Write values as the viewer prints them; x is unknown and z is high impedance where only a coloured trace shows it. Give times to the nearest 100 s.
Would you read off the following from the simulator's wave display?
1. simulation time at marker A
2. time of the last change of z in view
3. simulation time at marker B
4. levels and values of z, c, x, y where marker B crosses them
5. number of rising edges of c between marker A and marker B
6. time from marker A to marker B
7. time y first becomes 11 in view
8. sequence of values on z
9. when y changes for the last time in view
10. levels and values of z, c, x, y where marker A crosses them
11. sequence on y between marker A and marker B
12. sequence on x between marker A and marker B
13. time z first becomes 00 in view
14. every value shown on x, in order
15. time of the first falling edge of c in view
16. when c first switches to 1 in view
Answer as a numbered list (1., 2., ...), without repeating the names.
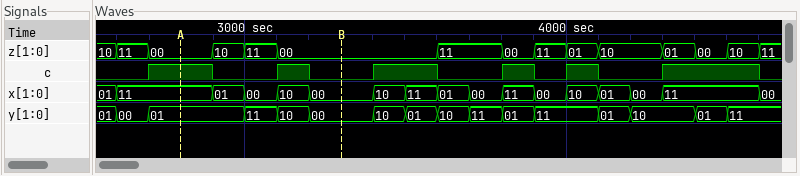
1. 2800 s
2. 4600 s
3. 3300 s
4. z=00, c=0, x=00, y=00
5. 1
6. 500 s
7. 3000 s
8. 10, 11, 00, 10, 11, 00, 11, 00, 11, 01, 10, 01, 00, 10, 11
9. 4500 s
10. z=00, c=1, x=11, y=01
11. 01, 11, 10, 00
12. 11, 01, 00, 10, 00
13. 2700 s
14. 01, 11, 01, 00, 10, 00, 10, 11, 01, 00, 11, 00, 10, 01, 00, 11, 00
15. 2900 s
16. 2700 s
